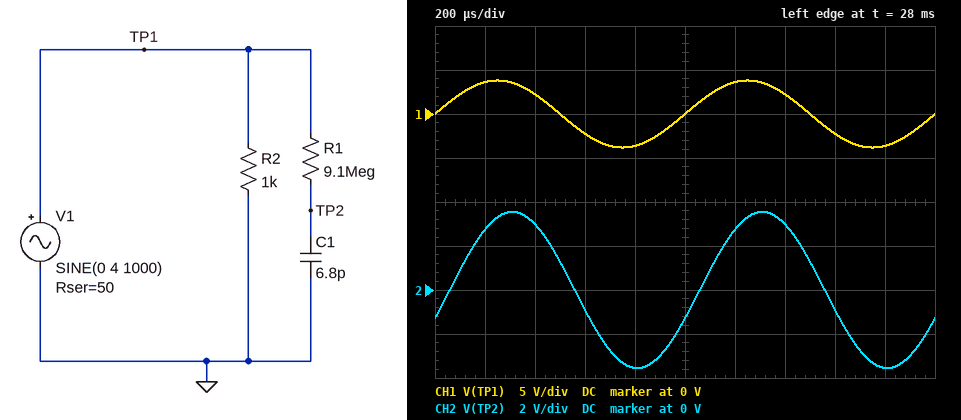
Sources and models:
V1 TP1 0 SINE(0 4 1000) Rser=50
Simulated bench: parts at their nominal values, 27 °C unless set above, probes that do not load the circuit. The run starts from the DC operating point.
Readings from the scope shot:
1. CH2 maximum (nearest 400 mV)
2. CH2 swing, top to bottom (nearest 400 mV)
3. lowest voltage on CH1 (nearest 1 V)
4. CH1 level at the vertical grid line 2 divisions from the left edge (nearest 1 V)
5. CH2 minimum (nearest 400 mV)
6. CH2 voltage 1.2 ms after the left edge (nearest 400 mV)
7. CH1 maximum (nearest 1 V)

3.6 V
7.2 V
-4 V
2 V
-3.6 V
2.8 V
4 V
